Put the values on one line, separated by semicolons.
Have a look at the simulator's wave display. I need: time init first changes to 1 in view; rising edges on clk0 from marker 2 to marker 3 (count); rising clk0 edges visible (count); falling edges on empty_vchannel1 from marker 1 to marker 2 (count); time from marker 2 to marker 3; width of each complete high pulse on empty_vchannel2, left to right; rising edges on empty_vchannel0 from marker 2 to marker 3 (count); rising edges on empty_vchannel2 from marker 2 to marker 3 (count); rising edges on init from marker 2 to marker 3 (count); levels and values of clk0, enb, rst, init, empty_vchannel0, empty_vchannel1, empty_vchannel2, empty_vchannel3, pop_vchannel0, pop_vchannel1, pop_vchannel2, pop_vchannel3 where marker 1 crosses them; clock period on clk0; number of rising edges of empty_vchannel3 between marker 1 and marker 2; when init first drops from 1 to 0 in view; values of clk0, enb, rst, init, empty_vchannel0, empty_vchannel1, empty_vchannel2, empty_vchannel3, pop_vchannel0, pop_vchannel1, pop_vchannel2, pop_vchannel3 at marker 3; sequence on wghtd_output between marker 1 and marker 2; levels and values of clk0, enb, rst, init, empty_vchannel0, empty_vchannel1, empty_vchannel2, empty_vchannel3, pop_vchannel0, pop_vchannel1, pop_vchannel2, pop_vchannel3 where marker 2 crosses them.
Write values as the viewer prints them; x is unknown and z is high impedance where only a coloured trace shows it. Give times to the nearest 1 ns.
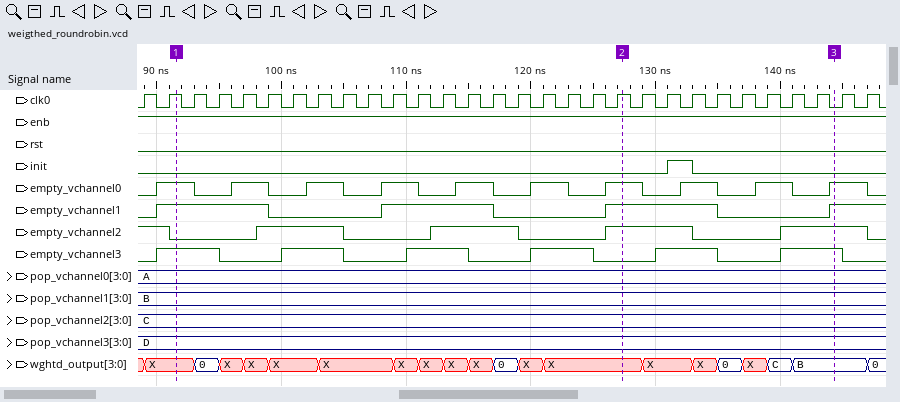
131 ns; 8; 30; 2; 17 ns; 7 ns, 7 ns, 7 ns, 7 ns; 3; 1; 1; clk0=1, enb=1, rst=0, init=0, empty_vchannel0=1, empty_vchannel1=1, empty_vchannel2=0, empty_vchannel3=1, pop_vchannel0=A, pop_vchannel1=B, pop_vchannel2=C, pop_vchannel3=D; 2 ns; 3; 133 ns; clk0=0, enb=1, rst=0, init=0, empty_vchannel0=1, empty_vchannel1=1, empty_vchannel2=1, empty_vchannel3=1, pop_vchannel0=A, pop_vchannel1=B, pop_vchannel2=C, pop_vchannel3=D; X, 0, X, X, X, X, X, X, X, X, 0, X, X; clk0=1, enb=1, rst=0, init=0, empty_vchannel0=1, empty_vchannel1=1, empty_vchannel2=1, empty_vchannel3=0, pop_vchannel0=A, pop_vchannel1=B, pop_vchannel2=C, pop_vchannel3=D
